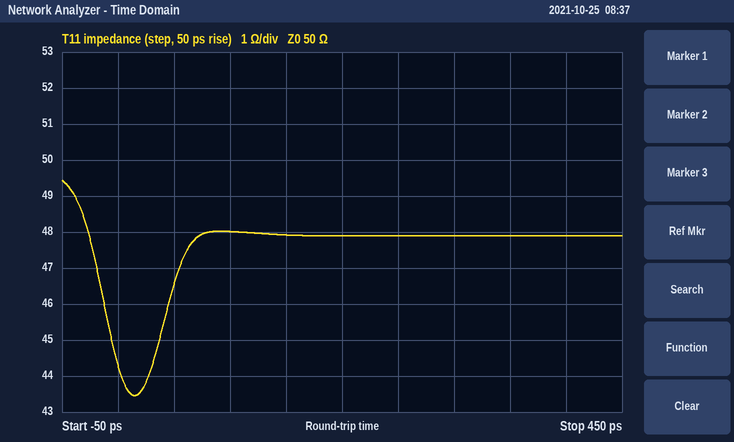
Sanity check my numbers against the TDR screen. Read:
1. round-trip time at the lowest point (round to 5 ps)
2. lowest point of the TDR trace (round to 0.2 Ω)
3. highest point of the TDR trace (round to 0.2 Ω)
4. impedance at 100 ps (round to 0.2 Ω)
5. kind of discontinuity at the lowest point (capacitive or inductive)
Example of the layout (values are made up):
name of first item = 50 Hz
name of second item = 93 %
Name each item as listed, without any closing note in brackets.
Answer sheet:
round-trip time at the lowest point = 15 ps
lowest point of the TDR trace = 43.4 Ω
highest point of the TDR trace = 49.4 Ω
impedance at 100 ps = 48.0 Ω
kind of discontinuity at the lowest point = capacitive
